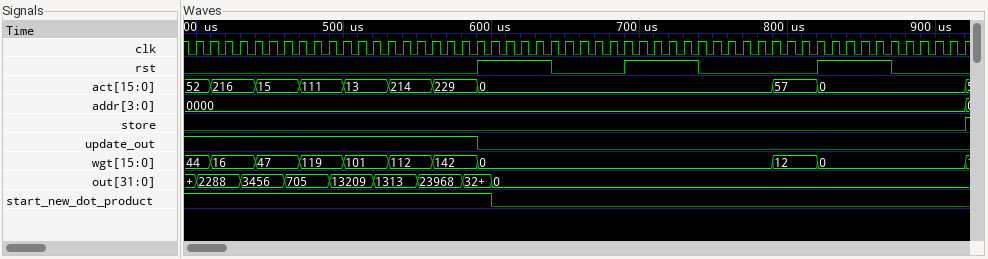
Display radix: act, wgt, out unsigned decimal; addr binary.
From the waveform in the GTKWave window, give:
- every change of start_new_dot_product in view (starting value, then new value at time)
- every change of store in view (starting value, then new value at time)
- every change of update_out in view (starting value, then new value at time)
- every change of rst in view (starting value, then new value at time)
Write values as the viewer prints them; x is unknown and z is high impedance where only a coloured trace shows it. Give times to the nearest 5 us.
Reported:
1, 0 at 600 us
0, 1 at 920 us
1, 0 at 590 us
0, 1 at 590 us, 0 at 640 us, 1 at 690 us, 0 at 740 us, 1 at 820 us, 0 at 870 us
